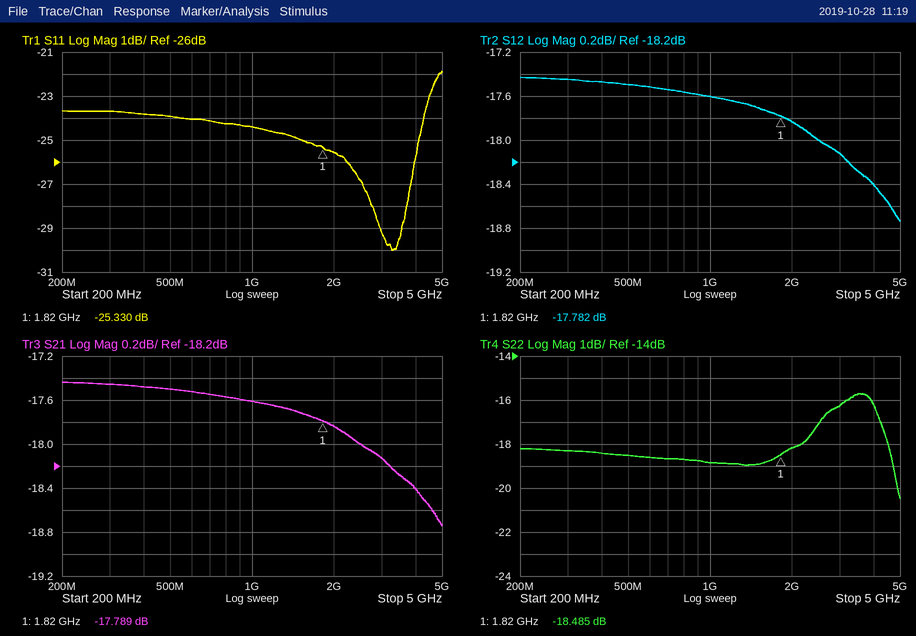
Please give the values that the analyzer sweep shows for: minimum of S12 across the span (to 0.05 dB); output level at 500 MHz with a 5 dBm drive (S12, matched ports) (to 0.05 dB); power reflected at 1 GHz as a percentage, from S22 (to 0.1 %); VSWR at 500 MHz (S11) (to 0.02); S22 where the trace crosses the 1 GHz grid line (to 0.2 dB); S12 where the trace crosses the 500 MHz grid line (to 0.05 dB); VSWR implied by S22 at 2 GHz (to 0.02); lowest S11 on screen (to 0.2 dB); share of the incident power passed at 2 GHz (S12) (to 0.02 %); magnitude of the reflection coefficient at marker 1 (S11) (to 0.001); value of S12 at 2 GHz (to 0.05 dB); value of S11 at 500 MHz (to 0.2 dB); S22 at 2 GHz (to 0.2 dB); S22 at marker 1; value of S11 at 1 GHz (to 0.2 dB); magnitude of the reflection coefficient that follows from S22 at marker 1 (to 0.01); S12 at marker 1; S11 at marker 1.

-18.75 dB
-12.50 dBm
1.3 %
1.14
-18.8 dB
-17.50 dB
1.28
-30.0 dB
1.64 %
0.054
-17.85 dB
-24.0 dB
-18.2 dB
-18.485 dB
-24.4 dB
0.12
-17.782 dB
-25.330 dB
